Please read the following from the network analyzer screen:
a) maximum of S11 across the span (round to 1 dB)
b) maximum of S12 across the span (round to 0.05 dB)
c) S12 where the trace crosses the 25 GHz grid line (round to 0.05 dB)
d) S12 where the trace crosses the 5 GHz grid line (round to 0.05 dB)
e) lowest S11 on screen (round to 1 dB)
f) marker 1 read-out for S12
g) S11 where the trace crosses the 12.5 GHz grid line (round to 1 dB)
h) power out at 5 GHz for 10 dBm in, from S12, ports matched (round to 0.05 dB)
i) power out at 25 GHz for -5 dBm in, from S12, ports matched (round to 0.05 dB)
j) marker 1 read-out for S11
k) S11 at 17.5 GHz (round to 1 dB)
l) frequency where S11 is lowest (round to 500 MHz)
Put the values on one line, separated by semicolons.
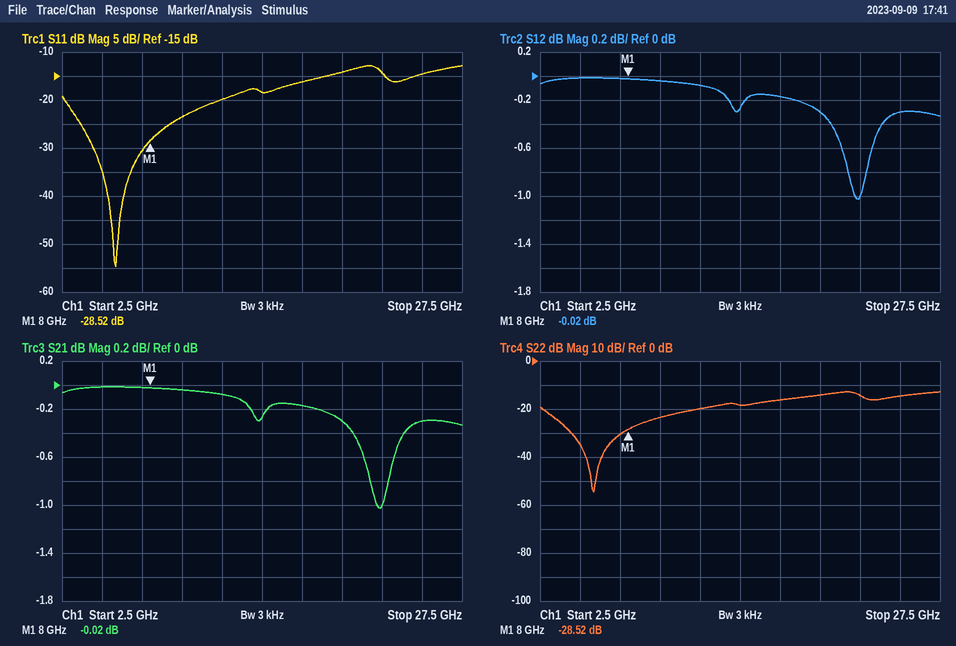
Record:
-13 dB; 0.00 dB; -0.30 dB; 0.00 dB; -55 dB; -0.02 dB; -20 dB; 10.00 dBm; -5.30 dBm; -28.52 dB; -16 dB; 6.0 GHz
